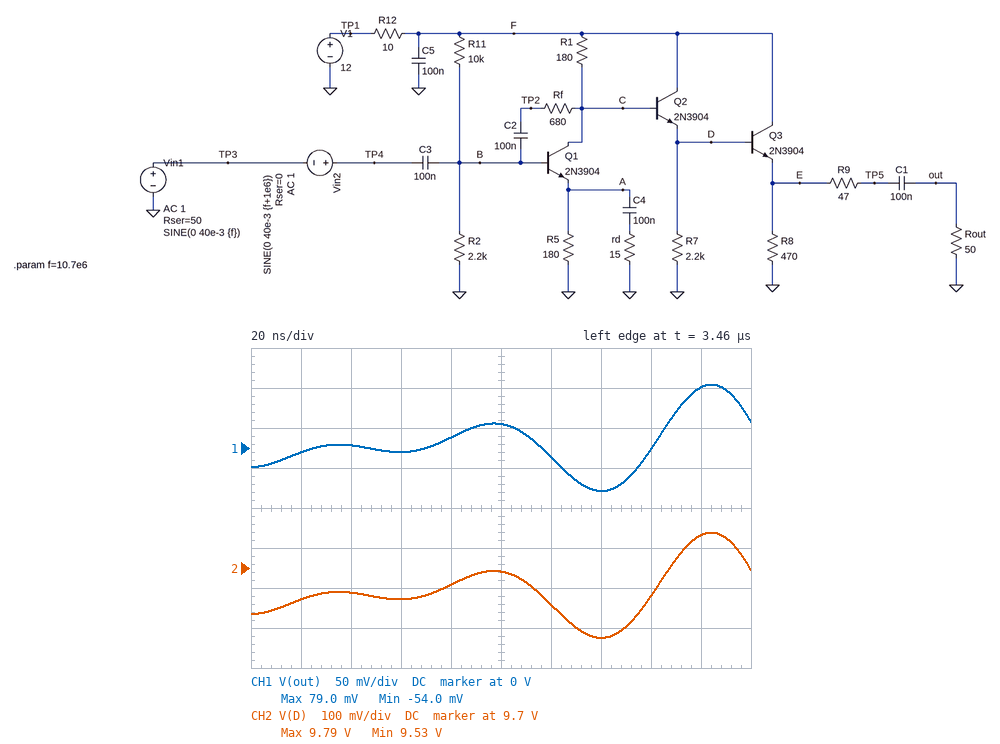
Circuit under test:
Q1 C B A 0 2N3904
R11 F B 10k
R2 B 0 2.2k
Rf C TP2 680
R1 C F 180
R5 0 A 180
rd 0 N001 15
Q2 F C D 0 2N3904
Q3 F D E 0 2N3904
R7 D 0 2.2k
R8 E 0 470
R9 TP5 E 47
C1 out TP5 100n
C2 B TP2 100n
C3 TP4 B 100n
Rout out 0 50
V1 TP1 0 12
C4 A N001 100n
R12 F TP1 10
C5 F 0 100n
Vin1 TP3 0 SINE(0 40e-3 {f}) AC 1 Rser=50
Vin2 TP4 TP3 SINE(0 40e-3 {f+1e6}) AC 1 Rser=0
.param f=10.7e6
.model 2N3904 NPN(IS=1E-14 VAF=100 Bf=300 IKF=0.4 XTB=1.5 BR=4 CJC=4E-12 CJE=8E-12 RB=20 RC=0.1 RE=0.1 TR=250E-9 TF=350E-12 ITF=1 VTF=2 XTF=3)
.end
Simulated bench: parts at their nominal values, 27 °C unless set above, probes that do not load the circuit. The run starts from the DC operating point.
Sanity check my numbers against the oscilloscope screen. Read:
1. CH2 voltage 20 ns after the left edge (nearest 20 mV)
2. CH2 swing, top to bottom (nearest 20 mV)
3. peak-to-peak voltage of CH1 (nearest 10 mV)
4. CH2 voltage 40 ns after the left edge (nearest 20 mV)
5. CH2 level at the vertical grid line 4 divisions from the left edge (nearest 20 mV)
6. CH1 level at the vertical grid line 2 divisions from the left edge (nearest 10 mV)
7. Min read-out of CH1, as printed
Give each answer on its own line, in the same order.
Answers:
9.62 V
260 mV
130 mV
9.64 V
9.66 V
0 V
-54.0 mV
